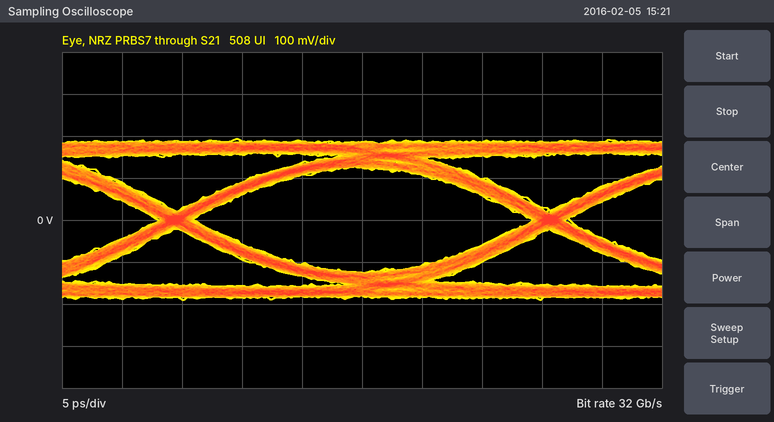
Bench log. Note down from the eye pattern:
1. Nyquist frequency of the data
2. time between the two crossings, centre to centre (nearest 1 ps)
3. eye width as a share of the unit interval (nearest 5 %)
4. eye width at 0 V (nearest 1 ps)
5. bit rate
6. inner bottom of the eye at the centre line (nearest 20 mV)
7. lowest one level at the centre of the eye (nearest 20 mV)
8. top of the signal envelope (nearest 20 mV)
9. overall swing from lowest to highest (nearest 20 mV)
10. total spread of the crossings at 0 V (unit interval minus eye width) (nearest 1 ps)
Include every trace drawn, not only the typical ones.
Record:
16 GHz
31 ps
90 %
28 ps
32 Gb/s
-120 mV
120 mV
200 mV
380 mV
3 ps
